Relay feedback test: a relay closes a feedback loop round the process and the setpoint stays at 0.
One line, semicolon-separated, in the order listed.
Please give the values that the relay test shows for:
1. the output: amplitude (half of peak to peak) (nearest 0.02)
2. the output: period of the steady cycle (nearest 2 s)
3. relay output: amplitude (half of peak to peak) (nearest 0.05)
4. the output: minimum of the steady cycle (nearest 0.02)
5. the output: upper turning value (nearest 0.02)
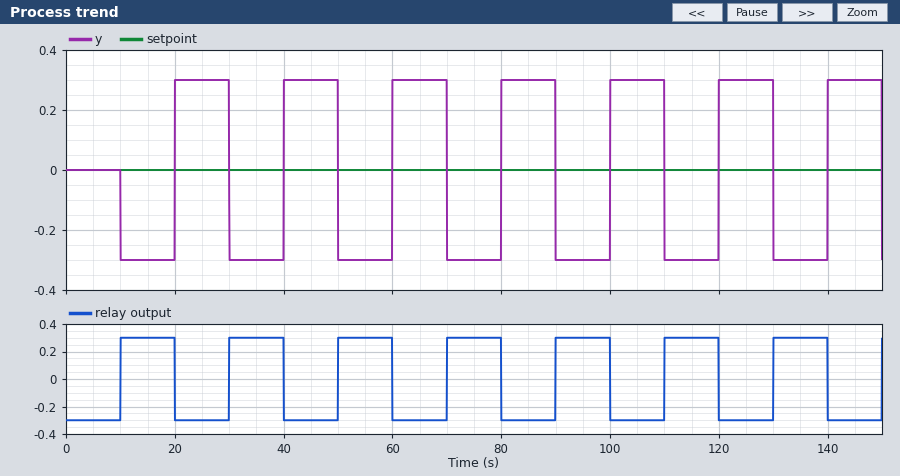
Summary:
0.30; 20 s; 0.30; -0.30; 0.30
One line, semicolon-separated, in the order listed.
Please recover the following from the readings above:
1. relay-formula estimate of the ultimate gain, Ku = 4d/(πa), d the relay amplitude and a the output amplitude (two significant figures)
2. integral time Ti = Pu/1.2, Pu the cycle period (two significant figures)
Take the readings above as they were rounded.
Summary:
1.3; 17 s
